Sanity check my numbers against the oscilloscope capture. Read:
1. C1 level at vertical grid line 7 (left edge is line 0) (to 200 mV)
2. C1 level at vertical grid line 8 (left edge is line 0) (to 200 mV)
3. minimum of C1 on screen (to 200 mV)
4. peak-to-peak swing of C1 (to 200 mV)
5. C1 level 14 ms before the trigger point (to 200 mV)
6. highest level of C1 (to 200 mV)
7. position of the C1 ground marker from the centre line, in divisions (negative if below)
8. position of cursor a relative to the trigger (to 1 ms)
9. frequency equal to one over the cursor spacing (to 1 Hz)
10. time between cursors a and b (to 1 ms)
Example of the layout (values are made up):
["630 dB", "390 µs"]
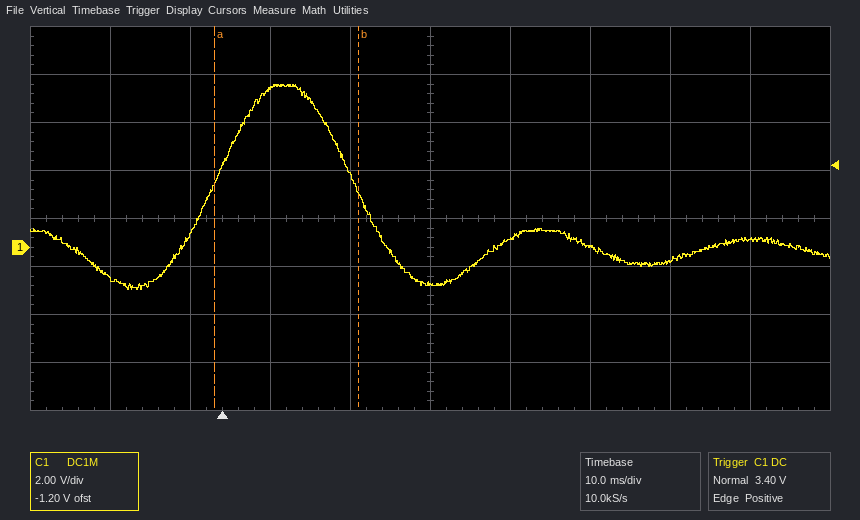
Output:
["0.0 V", "-600 mV", "-1.8 V", "8.6 V", "-1.2 V", "6.8 V", "-0.6 div", "-1 ms", "56 Hz", "18 ms"]
